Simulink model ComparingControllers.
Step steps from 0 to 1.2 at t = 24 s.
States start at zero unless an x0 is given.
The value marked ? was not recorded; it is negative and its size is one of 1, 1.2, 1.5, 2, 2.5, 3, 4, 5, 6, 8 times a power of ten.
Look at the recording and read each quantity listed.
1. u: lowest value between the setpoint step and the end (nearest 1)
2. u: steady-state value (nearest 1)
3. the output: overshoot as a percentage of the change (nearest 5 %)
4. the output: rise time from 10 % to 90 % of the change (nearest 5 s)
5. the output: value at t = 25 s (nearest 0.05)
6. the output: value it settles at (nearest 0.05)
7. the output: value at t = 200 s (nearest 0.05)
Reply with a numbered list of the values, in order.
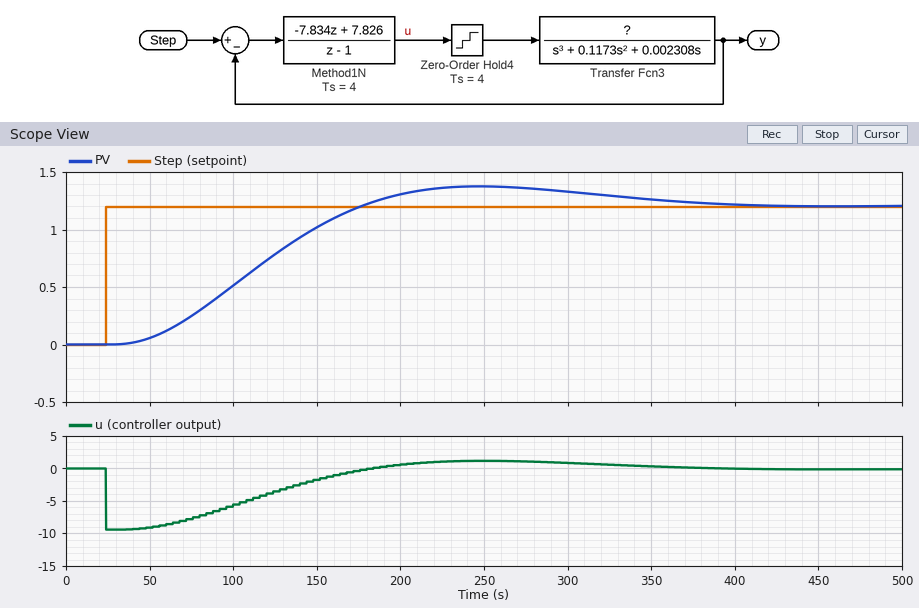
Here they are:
1. -9
2. 0
3. 15 %
4. 100 s
5. 0.00
6. 1.20
7. 1.30
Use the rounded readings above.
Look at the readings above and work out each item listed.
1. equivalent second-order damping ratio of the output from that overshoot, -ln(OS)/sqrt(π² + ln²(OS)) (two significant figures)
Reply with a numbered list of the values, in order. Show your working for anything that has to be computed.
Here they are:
1. ln(0.15) = -1.897; 1.897 / sqrt(9.870 + 3.599) = 0.52
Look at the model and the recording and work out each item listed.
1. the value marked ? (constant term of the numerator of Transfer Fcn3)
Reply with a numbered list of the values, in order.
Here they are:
1. -4e-06
